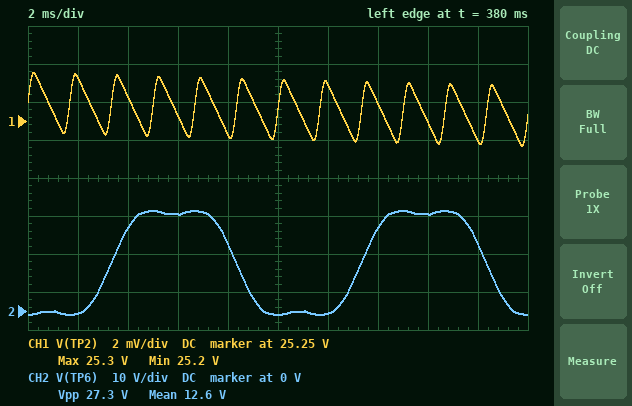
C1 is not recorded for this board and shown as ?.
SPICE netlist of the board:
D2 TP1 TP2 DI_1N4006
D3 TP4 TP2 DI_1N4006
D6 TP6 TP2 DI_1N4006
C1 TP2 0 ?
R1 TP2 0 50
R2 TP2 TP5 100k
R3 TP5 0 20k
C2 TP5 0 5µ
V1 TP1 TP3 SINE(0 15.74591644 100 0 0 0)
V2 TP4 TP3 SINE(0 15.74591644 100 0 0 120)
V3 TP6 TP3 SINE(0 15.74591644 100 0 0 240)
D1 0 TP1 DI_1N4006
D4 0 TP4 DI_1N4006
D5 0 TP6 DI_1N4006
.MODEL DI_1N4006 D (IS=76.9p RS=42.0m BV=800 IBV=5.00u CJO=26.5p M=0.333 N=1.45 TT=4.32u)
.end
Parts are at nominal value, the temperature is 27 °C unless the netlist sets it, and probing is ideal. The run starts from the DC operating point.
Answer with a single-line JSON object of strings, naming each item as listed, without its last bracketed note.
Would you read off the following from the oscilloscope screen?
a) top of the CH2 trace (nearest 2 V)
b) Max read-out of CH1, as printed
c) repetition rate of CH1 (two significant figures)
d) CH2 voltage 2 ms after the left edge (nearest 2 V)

{"top of the CH2 trace": "26 V", "Max read-out of CH1, as printed": "25.3 V", "repetition rate of CH1": "600 Hz", "CH2 voltage 2 ms after the left edge": "0 V"}
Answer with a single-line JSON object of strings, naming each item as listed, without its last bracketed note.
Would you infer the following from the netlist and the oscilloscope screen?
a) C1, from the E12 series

{"C1, from the E12 series": "180 mF"}
